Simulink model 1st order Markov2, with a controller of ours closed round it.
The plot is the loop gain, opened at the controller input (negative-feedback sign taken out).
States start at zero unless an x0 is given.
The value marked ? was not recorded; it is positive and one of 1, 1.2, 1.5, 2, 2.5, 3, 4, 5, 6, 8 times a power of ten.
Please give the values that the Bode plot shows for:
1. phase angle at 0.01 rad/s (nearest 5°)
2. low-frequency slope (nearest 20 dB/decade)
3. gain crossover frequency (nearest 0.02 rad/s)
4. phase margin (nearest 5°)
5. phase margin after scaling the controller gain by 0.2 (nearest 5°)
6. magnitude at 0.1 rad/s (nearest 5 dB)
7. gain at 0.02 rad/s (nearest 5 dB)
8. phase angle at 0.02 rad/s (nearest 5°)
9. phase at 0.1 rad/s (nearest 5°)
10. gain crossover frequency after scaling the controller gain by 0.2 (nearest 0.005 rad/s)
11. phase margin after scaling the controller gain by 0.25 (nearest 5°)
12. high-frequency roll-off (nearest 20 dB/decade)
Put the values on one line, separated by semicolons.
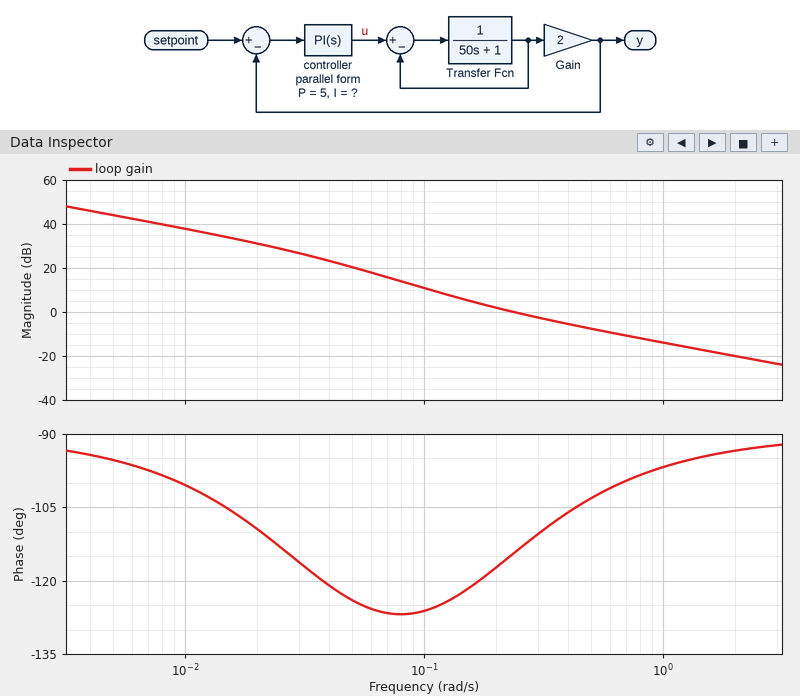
-100°; -20 dB/decade; 0.24 rad/s; 65°; 55°; 10 dB; 30 dB; -110°; -125°; 0.080 rad/s; 55°; -20 dB/decade
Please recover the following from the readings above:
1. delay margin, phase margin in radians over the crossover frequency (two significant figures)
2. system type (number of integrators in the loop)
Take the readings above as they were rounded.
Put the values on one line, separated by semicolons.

4.7 s; 1
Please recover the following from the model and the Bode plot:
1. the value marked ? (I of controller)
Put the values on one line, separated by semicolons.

0.8
